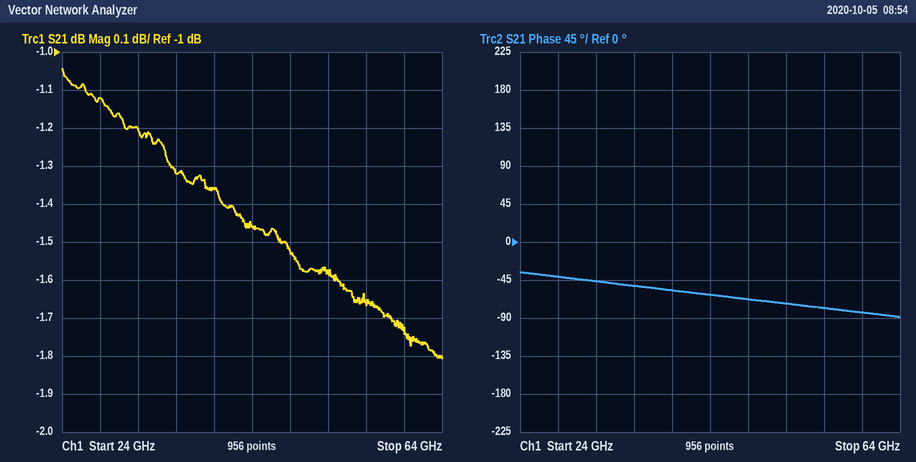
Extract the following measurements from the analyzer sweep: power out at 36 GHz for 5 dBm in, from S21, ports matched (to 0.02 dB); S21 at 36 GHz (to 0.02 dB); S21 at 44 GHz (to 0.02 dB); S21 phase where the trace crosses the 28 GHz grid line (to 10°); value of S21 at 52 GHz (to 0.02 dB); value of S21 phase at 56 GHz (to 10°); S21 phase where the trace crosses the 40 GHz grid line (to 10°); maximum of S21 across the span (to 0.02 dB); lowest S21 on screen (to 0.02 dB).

3.68 dBm
-1.32 dB
-1.46 dB
-40°
-1.58 dB
-80°
-60°
-1.04 dB
-1.80 dB
